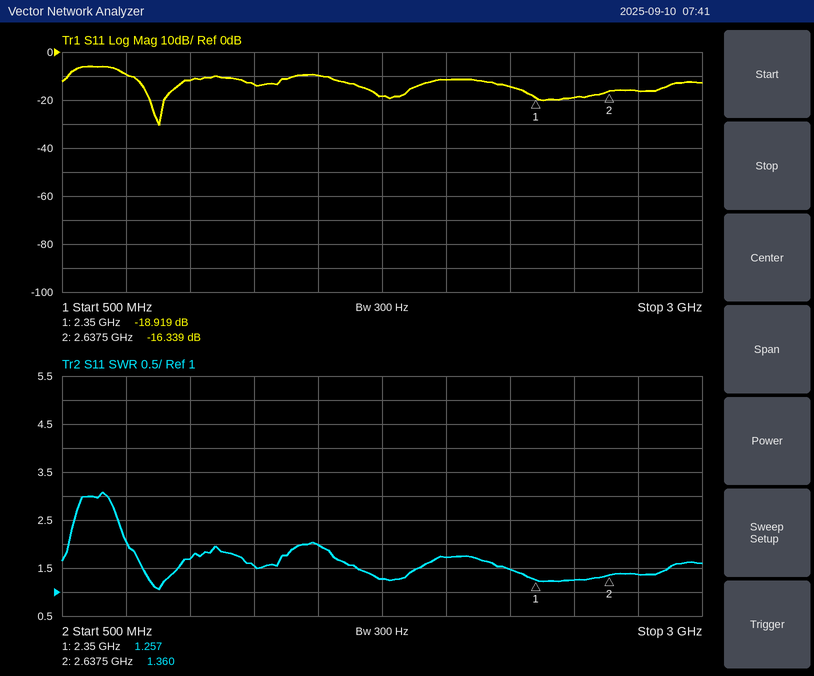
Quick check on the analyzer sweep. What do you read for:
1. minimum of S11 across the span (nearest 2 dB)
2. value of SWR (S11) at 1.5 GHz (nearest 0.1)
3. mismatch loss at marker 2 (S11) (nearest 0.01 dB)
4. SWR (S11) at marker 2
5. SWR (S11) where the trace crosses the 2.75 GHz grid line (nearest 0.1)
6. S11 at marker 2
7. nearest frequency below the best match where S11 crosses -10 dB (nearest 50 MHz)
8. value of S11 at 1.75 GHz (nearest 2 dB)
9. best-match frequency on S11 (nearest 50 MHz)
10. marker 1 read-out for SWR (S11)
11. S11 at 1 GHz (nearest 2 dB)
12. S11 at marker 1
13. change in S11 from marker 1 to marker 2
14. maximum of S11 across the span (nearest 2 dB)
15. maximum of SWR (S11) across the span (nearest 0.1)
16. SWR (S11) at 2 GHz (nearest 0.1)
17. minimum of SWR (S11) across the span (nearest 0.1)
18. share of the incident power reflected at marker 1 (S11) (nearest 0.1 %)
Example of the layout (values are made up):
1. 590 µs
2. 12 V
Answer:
1. -30 dB
2. 2.0
3. 0.10 dB
4. 1.360
5. 1.4
6. -16.339 dB
7. 750 MHz
8. -18 dB
9. 900 MHz
10. 1.257
11. -12 dB
12. -18.919 dB
13. 2.580 dB
14. -6 dB
15. 3.1
16. 1.7
17. 1.1
18. 1.3 %
